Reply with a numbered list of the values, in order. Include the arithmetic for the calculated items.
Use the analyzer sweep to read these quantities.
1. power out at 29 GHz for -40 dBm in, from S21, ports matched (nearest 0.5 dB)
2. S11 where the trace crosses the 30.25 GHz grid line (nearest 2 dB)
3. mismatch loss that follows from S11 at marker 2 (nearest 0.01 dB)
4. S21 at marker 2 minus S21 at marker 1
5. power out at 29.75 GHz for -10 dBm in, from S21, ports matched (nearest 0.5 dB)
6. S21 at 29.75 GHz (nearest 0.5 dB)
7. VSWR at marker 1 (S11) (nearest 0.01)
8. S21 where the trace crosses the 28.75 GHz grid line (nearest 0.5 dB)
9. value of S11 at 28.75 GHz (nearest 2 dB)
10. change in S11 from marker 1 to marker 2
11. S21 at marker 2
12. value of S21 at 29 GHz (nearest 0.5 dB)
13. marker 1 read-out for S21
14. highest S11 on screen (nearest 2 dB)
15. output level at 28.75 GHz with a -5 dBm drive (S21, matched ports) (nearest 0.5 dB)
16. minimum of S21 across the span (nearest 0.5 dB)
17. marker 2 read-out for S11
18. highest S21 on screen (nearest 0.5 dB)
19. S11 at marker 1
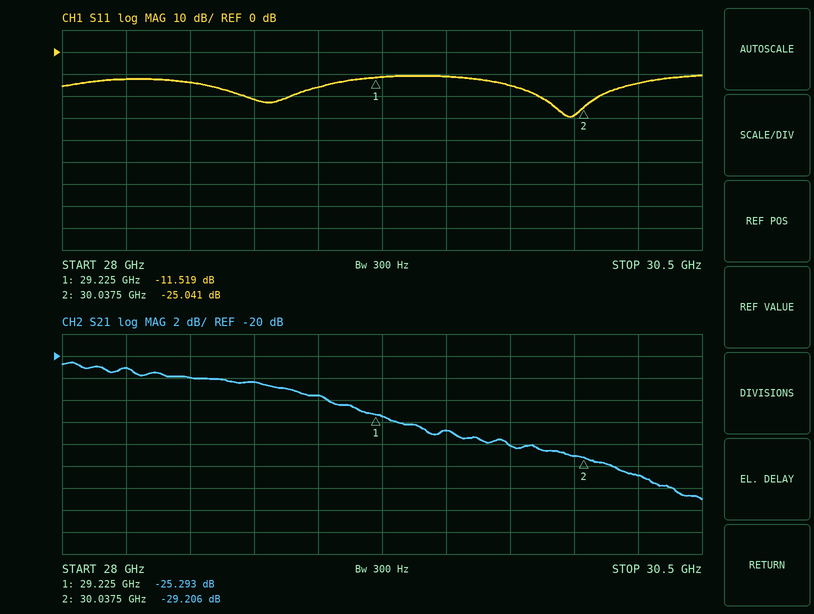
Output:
1. -40 dBm + (-23.5 dB) = -63.5 dBm
2. -14 dB
3. −10 log10(1 − 10^(-25.041/10)) ≈ 0.01 dB
4. -29.206 − (-25.293) = -3.913 dB
5. -10 dBm + (-28.0 dB) = -38.0 dBm
6. -28.0 dB
7. (1 + 0.2655)/(1 − 0.2655) ≈ 1.72
8. -22.5 dB
9. -22 dB
10. -25.041 − (-11.519) = -13.522 dB
11. -29.206 dB
12. -23.5 dB
13. -25.293 dB
14. -10 dB
15. -5 dBm + (-22.5 dB) = -27.5 dBm
16. -33.0 dB
17. -25.041 dB
18. -20.5 dB
19. -11.519 dB
